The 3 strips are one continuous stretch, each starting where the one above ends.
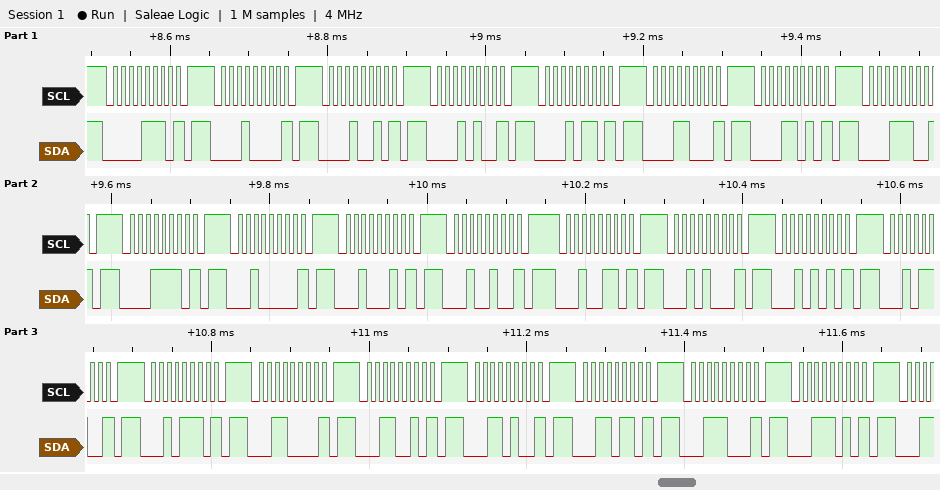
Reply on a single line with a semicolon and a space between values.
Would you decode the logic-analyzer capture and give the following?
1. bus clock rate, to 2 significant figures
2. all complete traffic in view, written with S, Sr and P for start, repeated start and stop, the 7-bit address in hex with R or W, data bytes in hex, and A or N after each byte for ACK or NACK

100 kHz; S 07W N P S 08W N P S 09W N P S 0AW N P S 0BW N P S 0CW N P S 0DW N P S 0EW N P S 0FW N P S 10W N P S 11W N P S 12W N P S 13W N P S 14W N P S 15W N P S 16W N P S 17W N P S 18W N P S 19W N P S 1AW N P S 1BW N P S 1CW N P S 1DW N P
